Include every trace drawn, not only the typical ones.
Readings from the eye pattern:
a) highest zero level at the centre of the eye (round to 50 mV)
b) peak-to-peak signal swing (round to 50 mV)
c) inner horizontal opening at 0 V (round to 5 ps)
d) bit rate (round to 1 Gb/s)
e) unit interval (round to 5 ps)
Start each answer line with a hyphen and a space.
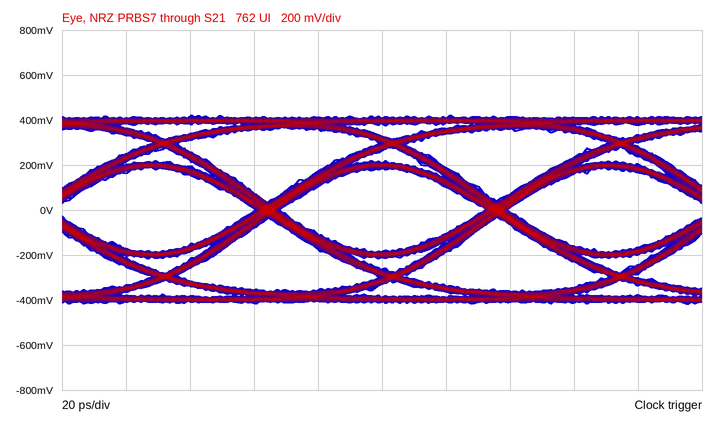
- -200 mV
- 850 mV
- 65 ps
- 14 Gb/s
- 70 ps
